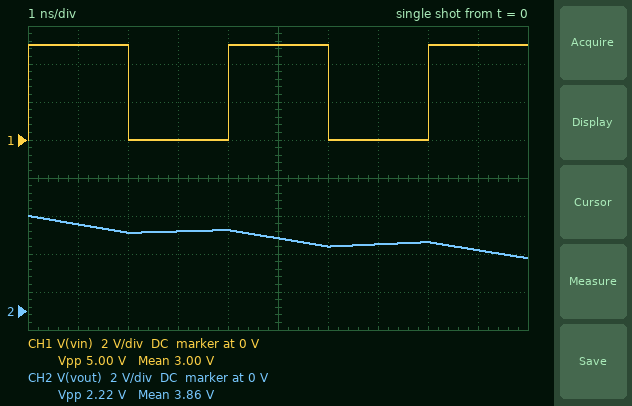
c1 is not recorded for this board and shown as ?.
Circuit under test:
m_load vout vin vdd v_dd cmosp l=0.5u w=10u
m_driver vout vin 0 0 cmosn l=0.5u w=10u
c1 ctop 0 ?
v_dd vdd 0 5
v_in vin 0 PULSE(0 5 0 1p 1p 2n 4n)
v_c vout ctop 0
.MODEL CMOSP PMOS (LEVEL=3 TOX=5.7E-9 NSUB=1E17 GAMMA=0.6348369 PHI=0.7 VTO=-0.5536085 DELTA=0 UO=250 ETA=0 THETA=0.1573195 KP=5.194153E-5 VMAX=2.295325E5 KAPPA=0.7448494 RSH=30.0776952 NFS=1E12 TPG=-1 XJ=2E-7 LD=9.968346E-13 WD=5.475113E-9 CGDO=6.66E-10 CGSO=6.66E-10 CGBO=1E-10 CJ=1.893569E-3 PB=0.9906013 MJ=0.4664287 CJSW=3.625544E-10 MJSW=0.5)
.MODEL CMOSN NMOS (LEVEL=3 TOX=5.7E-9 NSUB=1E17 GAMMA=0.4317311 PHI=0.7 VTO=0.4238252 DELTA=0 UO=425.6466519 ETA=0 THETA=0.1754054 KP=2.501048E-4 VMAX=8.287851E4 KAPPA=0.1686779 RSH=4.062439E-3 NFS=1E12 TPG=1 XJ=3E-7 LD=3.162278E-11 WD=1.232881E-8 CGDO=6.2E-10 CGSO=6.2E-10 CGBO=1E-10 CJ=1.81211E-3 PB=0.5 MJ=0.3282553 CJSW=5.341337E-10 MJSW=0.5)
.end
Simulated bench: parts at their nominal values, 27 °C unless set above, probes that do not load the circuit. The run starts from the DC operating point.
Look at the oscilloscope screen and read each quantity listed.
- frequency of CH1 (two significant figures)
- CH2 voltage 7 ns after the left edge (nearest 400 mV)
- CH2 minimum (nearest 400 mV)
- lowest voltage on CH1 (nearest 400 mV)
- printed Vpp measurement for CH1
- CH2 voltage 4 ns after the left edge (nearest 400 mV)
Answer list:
250 MHz
3.6 V
2.8 V
0 V
5.00 V
4.4 V
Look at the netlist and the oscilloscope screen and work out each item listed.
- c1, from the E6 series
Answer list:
22 pF
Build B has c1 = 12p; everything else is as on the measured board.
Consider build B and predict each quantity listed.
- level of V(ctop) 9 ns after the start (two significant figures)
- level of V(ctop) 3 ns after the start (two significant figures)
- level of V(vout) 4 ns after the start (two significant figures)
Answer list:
2.1 V
3.6 V
3.8 V
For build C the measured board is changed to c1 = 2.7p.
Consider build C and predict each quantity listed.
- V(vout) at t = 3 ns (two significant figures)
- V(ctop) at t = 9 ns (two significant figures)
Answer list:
1.4 V
190 mV
